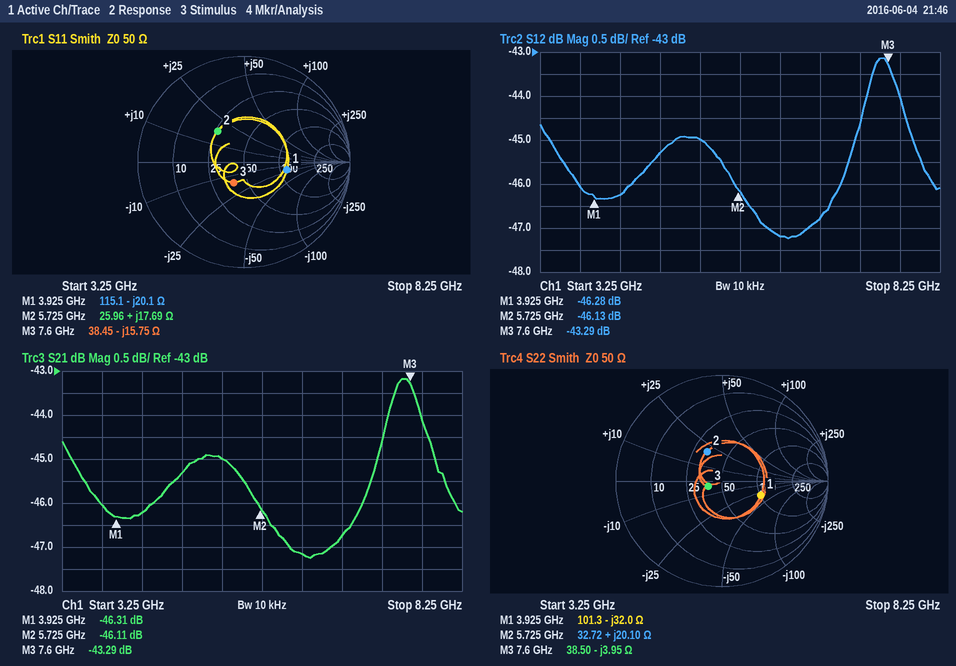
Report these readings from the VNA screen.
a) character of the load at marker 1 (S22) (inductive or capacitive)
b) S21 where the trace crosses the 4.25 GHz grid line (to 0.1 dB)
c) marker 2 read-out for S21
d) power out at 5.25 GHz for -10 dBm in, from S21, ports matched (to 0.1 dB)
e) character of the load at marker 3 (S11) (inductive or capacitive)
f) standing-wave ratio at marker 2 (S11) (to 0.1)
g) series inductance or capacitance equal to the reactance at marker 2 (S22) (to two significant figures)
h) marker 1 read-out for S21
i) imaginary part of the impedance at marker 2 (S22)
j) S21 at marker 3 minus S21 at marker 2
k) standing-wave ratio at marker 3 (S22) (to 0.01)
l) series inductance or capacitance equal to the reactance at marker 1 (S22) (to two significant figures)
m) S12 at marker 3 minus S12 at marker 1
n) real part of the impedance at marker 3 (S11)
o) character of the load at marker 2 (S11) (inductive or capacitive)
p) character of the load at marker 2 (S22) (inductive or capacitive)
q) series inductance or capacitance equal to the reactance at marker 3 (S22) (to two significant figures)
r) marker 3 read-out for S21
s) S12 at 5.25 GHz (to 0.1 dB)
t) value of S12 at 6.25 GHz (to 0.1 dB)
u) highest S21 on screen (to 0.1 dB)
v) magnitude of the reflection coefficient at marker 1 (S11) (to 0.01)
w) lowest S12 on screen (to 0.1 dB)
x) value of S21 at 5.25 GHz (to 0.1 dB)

capacitive
-46.2 dB
-46.11 dB
-55.0 dBm
capacitive
2.2
560 pH
-46.31 dB
+20.10 Ω
2.82 dB
1.32
1.3 pF
2.99 dB
38.45 Ω
inductive
inductive
5.3 pF
-43.29 dB
-45.0 dB
-47.2 dB
-43.2 dB
0.41
-47.2 dB
-45.0 dB
